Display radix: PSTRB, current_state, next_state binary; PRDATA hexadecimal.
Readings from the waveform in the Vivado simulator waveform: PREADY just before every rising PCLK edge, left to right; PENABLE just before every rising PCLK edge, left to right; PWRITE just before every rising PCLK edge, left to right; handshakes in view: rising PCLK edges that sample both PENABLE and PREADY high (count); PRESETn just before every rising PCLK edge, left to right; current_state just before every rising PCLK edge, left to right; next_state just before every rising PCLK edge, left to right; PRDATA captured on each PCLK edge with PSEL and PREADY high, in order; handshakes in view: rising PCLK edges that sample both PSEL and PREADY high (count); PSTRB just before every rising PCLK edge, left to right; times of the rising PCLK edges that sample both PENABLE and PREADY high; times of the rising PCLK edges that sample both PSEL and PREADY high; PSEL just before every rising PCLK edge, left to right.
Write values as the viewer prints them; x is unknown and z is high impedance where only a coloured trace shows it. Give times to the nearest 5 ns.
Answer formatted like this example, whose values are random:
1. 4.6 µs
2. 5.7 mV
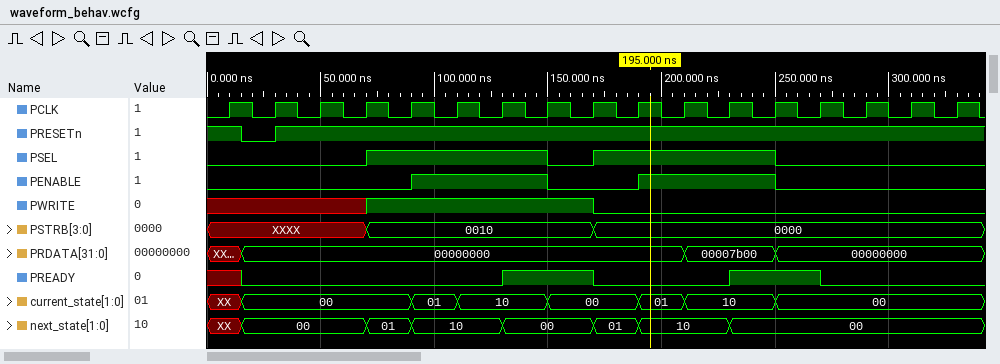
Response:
1. x 0 0 0 0 0 0 1 1 0 0 0 1 1 0 0 0
2. 0 0 0 0 0 1 1 1 0 0 1 1 1 0 0 0 0
3. x x x x 1 1 1 1 1 0 0 0 0 0 0 0 0
4. 2
5. 1 0 1 1 1 1 1 1 1 1 1 1 1 1 1 1 1
6. XX, 00, 00, 00, 00, 01, 10, 10, 00, 00, 01, 10, 10, 00, 00, 00, 00
7. XX, 00, 00, 00, 01, 10, 10, 00, 00, 01, 10, 10, 00, 00, 00, 00, 00
8. 00000000, 00007b00
9. 2
10. XXXX, XXXX, XXXX, XXXX, 0010, 0010, 0010, 0010, 0010, 0000, 0000, 0000, 0000, 0000, 0000, 0000, 0000
11. 150 ns, 250 ns
12. 150 ns, 250 ns
13. 0 0 0 0 1 1 1 1 0 1 1 1 1 0 0 0 0
